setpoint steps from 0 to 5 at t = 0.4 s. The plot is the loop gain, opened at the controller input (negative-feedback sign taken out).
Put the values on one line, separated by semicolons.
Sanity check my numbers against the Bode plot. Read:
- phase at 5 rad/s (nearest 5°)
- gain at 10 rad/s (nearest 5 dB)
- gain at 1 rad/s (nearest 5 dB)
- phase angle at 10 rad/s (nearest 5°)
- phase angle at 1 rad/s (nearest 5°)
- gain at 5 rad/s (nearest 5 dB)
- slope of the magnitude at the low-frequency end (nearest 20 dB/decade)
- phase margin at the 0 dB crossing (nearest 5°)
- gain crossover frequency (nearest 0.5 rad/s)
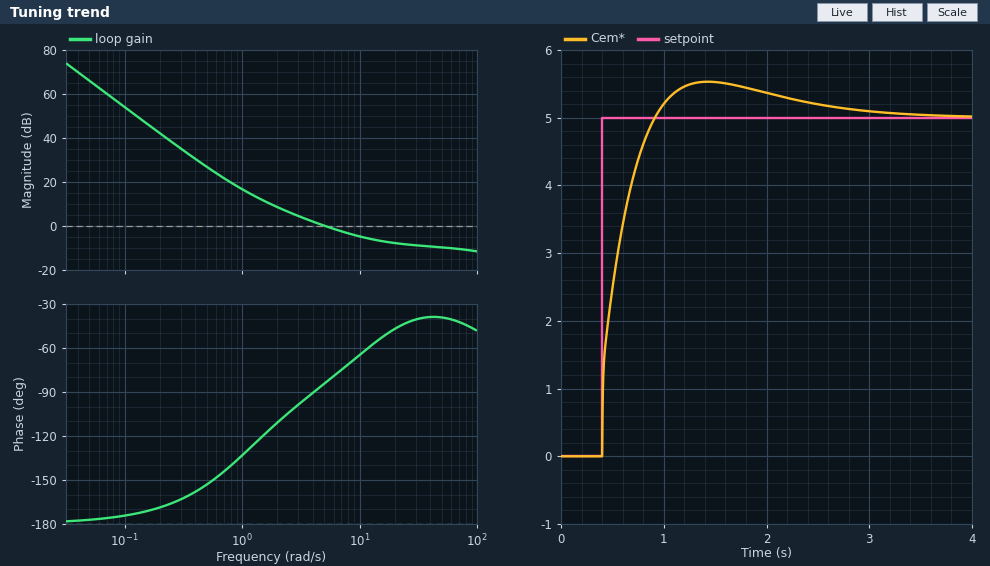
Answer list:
-85°; -5 dB; 15 dB; -65°; -135°; 0 dB; -40 dB/decade; 95°; 5.0 rad/s
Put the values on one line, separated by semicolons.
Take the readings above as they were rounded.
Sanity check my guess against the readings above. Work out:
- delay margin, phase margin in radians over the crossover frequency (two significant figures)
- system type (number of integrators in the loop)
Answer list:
0.33 s; 2
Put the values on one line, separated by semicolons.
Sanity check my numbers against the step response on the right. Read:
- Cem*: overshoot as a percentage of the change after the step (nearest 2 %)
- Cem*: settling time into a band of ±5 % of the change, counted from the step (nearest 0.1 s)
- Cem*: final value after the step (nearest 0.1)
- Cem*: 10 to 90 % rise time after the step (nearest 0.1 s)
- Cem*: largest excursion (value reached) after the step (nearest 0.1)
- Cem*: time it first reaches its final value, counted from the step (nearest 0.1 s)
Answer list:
10 %; 1.9 s; 5.0; 0.4 s; 5.5; 0.5 s
